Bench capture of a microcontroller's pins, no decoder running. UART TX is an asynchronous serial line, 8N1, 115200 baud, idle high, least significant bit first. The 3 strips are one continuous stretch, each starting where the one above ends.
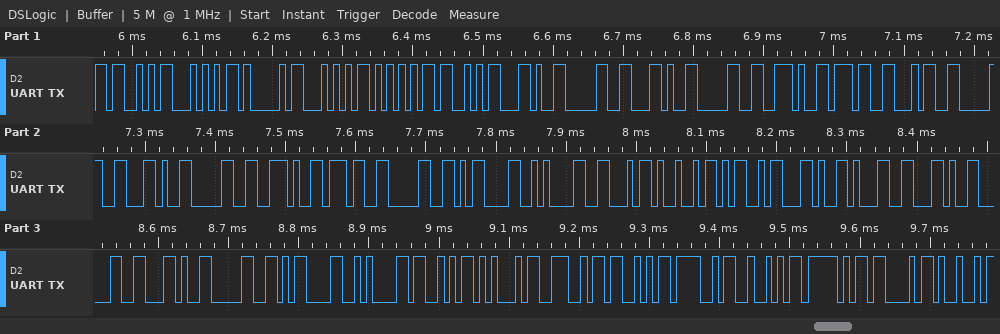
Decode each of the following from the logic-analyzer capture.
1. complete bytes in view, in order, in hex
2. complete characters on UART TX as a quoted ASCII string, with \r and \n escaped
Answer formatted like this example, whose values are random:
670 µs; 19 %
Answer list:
53 54 41 54 55 53 2C 30 2C 30 2E 37 34 30 2C 30 2E 37 30 0D 0A 46 49 4D 2C 31 2C 30 2C 30 0D 0A 53 45 4E 53 4F 52 5F 43 49; "STATUS,0,0.740,0.70\r\nFIM,1,0,0\r\nSENSOR_CI"
